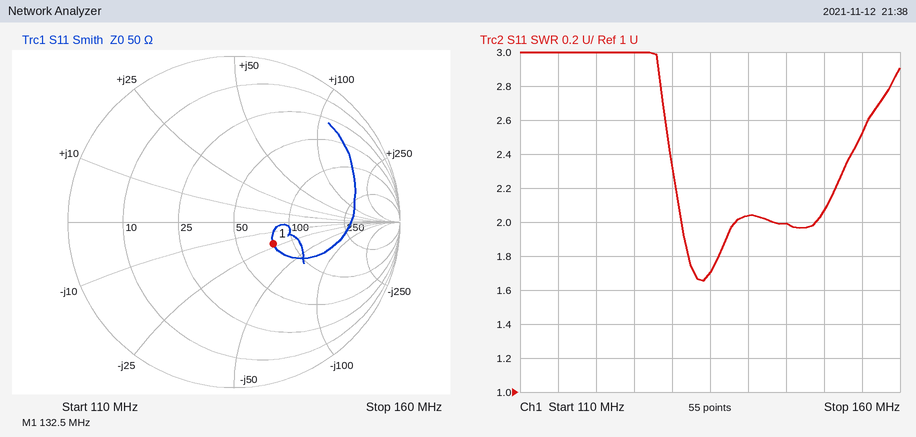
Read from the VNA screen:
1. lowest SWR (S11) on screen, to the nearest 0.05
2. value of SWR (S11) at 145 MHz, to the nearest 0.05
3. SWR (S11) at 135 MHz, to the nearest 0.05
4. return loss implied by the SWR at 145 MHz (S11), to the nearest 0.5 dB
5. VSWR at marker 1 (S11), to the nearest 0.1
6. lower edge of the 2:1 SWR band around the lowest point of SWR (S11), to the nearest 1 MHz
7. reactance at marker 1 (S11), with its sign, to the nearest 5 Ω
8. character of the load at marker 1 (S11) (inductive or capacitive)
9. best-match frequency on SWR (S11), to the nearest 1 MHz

1.65
2.00
1.70
9.5 dB
1.7
131 MHz
-20 Ω
capacitive
134 MHz
